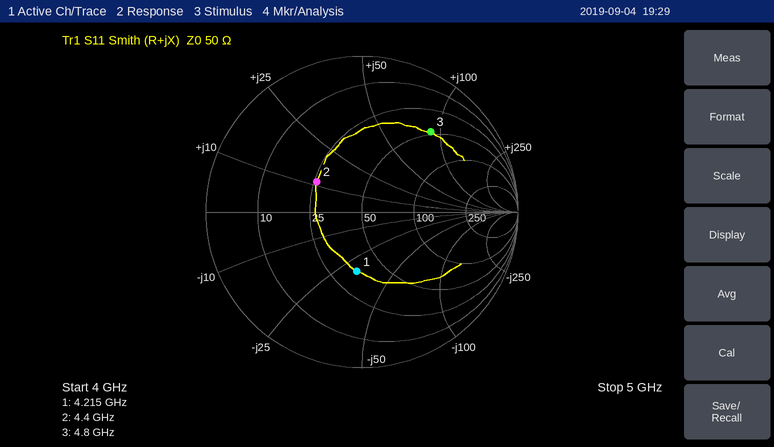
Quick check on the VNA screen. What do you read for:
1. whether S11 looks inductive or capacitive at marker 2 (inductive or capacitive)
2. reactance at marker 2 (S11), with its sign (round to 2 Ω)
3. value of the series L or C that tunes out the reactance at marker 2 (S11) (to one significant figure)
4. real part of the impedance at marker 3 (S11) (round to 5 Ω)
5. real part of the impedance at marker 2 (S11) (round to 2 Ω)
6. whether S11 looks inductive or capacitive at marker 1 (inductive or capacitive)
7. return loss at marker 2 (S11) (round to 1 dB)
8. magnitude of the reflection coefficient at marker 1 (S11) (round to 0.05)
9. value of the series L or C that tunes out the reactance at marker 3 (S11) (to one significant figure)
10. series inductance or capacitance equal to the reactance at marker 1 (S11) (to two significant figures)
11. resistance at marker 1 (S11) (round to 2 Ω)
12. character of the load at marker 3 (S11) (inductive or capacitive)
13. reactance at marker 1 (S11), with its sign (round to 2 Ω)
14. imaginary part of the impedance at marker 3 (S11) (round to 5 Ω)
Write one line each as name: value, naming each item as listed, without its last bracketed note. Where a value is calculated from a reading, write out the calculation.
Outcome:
whether S11 looks inductive or capacitive at marker 2: inductive
reactance at marker 2 (S11), with its sign: +12 Ω
value of the series L or C that tunes out the reactance at marker 2 (S11): C = 1/(2π × 4.4 GHz × 12 Ω) ≈ 3 pF
real part of the impedance at marker 3 (S11): 45 Ω
real part of the impedance at marker 2 (S11): 26 Ω
whether S11 looks inductive or capacitive at marker 1: capacitive
return loss at marker 2 (S11): 9 dB
magnitude of the reflection coefficient at marker 1 (S11): 0.40
value of the series L or C that tunes out the reactance at marker 3 (S11): C = 1/(2π × 4.8 GHz × 90 Ω) ≈ 368 fF, so 400 fF to one significant figure
series inductance or capacitance equal to the reactance at marker 1 (S11): C = 1/(2π × 4.215 GHz × 32 Ω) ≈ 1.2 pF
resistance at marker 1 (S11): 36 Ω
character of the load at marker 3 (S11): inductive
reactance at marker 1 (S11), with its sign: -32 Ω
imaginary part of the impedance at marker 3 (S11): +90 Ω
